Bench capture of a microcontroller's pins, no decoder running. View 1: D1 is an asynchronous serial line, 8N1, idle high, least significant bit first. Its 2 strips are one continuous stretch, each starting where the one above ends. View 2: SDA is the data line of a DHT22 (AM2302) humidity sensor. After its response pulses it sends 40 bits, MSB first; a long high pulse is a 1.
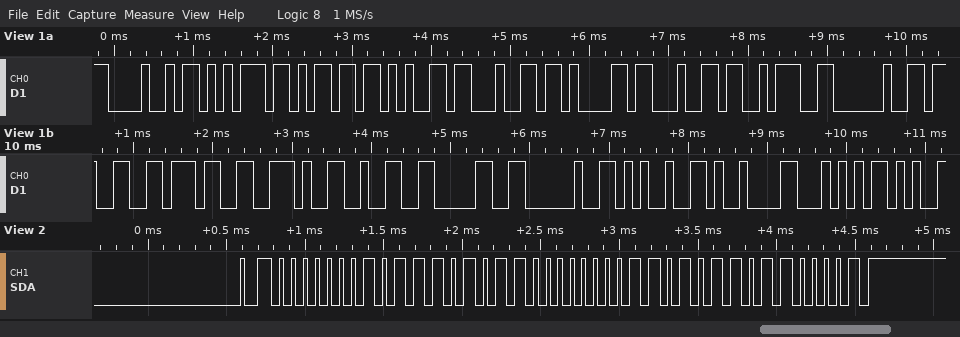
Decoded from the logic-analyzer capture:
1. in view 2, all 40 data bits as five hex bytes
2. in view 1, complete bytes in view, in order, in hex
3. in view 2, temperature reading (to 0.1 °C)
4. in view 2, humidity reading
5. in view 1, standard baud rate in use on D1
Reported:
01 75 80 6B 61
48 75 6D 65 64 61 64 3A 20 33 37 2E 32 30 20 25 09 54
-10.7 °C
37.3 %
9600 baud
